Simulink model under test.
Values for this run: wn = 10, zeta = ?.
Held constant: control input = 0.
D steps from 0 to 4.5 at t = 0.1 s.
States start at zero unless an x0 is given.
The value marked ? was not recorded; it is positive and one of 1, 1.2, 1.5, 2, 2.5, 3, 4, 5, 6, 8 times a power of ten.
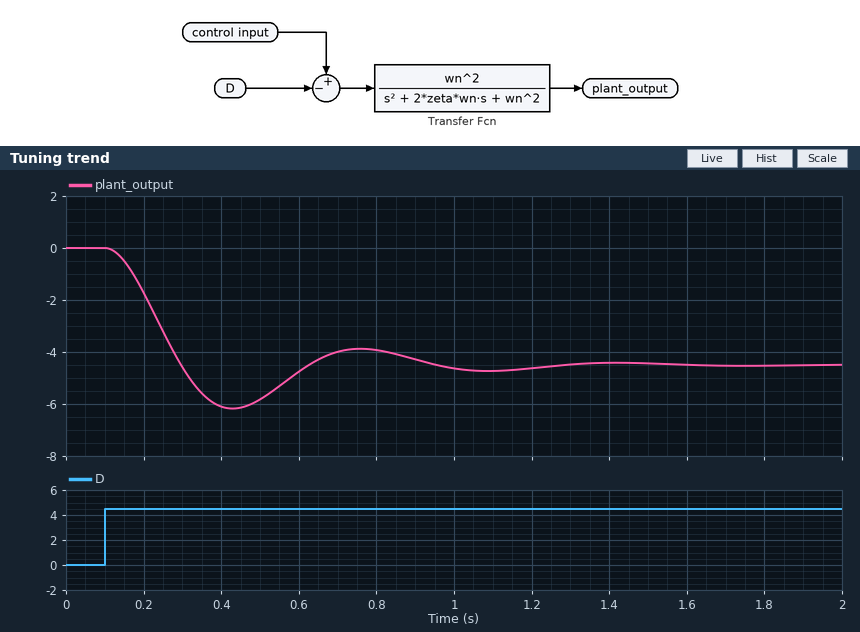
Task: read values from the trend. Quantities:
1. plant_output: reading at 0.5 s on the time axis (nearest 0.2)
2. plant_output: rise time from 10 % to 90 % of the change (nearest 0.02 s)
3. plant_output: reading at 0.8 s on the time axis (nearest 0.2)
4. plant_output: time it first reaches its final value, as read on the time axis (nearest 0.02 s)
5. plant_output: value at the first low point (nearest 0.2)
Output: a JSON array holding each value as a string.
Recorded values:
["-5.8", "0.14 s", "-4.0", "0.30 s", "-6.2"]
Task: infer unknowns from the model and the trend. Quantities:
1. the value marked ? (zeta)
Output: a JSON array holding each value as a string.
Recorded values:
["0.3"]
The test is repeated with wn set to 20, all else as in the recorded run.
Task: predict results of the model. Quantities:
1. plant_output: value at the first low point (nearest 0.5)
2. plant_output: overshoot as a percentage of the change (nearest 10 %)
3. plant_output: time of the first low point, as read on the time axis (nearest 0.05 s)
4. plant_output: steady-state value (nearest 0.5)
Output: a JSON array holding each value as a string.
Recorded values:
["-6.0", "40 %", "0.25 s", "-4.5"]
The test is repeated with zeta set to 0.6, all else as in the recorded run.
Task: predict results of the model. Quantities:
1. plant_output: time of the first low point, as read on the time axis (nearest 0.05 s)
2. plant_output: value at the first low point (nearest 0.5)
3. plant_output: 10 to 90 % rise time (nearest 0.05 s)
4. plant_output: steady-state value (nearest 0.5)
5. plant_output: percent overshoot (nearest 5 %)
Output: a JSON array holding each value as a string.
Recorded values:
["0.50 s", "-5.0", "0.20 s", "-4.5", "10 %"]
